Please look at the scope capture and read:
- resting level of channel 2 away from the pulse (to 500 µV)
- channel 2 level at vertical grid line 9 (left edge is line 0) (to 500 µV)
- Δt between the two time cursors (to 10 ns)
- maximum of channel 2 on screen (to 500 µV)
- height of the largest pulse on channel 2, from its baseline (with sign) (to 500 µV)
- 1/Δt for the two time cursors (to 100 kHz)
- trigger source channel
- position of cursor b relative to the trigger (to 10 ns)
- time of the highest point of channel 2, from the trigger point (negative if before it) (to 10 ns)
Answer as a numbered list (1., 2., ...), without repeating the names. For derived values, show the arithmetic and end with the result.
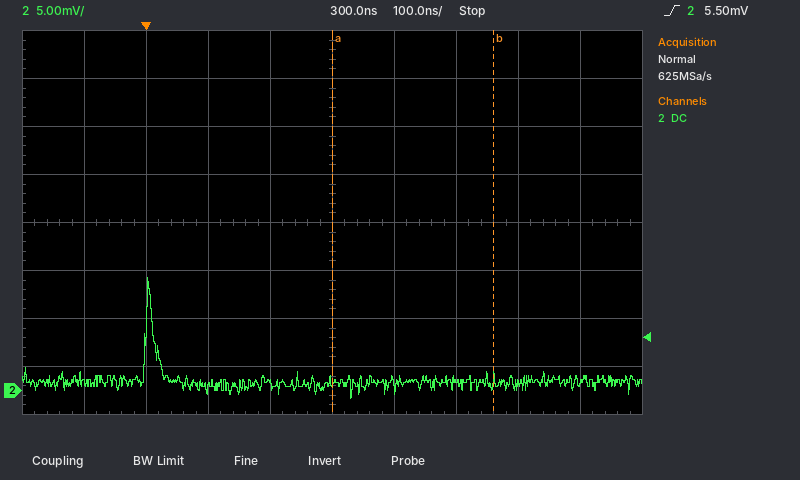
1. 1.0 mV
2. 1.0 mV
3. 260 ns
4. 12.0 mV
5. 12.0 mV − (1.0 mV) = +11.0 mV
6. 1 / 260 ns ≈ 3.8 MHz
7. channel 2
8. +560 ns
9. 0 ns
